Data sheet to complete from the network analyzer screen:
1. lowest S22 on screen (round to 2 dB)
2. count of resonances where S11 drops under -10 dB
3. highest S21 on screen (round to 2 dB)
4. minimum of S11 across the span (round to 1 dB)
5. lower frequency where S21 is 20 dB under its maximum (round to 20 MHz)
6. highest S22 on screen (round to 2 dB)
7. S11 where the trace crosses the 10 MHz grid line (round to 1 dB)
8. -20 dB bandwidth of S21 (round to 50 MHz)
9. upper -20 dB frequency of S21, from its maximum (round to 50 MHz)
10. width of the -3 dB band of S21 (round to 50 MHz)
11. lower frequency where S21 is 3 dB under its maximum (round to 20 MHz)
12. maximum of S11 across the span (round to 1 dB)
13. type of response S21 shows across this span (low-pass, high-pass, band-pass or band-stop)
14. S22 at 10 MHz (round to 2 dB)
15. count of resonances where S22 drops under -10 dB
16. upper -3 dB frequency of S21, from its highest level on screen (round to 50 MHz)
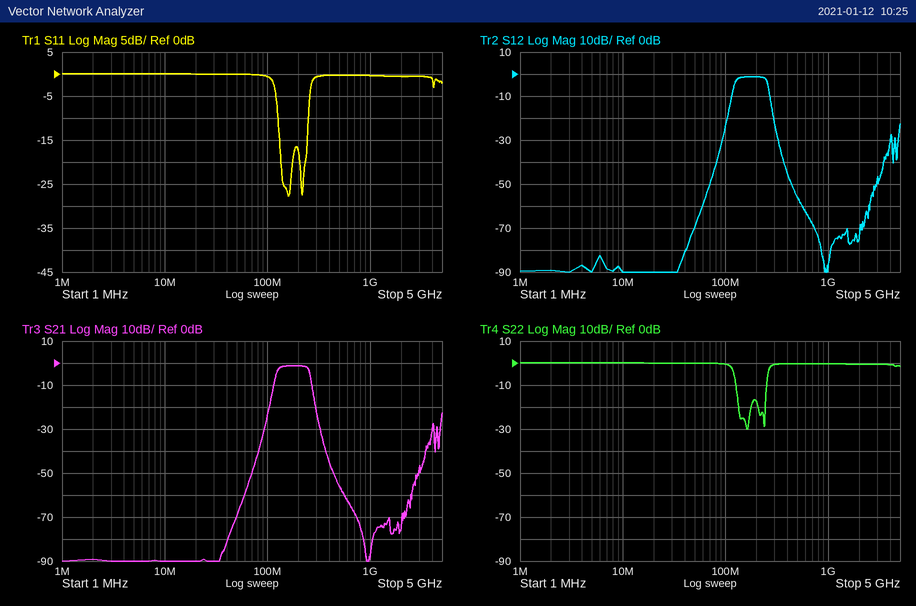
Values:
-30 dB
2
-2 dB
-28 dB
100 MHz
0 dB
0 dB
200 MHz
300 MHz
150 MHz
120 MHz
0 dB
band-pass
0 dB
2
250 MHz
